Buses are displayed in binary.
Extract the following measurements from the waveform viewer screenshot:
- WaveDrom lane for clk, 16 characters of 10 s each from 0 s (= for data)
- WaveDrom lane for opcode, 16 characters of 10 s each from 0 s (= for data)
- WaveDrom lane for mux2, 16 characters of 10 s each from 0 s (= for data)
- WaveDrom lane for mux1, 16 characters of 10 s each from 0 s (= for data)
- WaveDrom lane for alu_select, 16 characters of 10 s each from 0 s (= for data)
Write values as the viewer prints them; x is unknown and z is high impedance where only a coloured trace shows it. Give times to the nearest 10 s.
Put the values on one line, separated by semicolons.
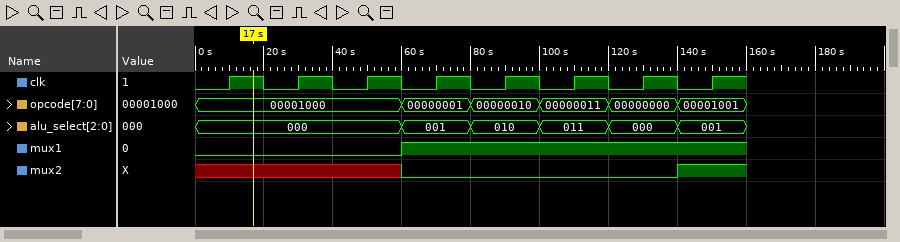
{name: 'clk', wave: '0101010101010101'}; {name: 'opcode', wave: '=.....=.=.=.=.=.', data: '00001000 00000001 00000010 00000011 00000000 00001001'}; {name: 'mux2', wave: 'x.....0.......1.'}; {name: 'mux1', wave: '0.....1.........'}; {name: 'alu_select', wave: '=.....=.=.=.=.=.', data: '000 001 010 011 000 001'}
